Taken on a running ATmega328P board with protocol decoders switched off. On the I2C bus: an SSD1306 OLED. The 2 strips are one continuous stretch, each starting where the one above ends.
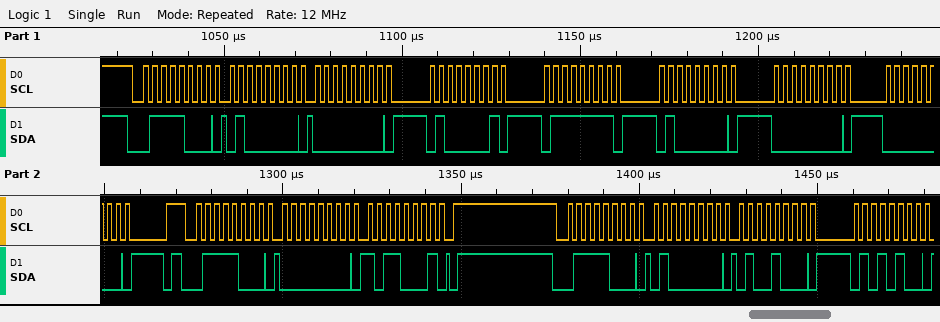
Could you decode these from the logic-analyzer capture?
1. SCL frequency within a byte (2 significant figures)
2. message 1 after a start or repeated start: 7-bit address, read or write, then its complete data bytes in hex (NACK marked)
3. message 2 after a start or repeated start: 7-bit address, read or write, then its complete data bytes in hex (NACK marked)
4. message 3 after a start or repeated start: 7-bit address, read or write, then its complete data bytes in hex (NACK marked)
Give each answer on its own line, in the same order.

400 kHz
0x3C write: 40 00 41 7F 40 00 00
0x3C write: 00 B1
0x3C write: 40 48 54
